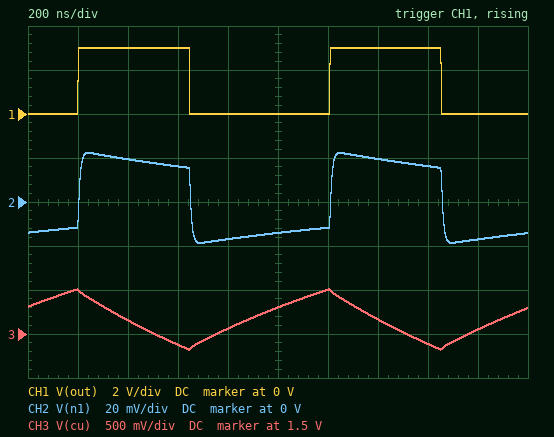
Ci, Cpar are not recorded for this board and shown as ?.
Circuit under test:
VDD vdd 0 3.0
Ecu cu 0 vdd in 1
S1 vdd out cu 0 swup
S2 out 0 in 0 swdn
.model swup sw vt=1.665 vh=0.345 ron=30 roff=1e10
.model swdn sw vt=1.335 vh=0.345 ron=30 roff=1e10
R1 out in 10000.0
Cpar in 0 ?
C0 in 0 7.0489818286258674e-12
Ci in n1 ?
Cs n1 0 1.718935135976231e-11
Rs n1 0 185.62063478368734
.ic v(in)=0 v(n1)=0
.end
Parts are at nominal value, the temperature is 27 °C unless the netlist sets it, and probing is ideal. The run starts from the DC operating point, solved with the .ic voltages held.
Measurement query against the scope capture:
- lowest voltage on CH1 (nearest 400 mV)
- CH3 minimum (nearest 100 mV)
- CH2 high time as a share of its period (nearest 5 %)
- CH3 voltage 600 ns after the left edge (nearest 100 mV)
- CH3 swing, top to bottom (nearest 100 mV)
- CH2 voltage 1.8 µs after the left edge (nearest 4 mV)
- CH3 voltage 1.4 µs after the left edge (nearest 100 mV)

0 V
1.3 V
45 %
1.4 V
700 mV
-16 mV
1.7 V
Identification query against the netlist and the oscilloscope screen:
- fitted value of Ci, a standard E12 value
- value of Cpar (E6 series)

68 pF
33 pF
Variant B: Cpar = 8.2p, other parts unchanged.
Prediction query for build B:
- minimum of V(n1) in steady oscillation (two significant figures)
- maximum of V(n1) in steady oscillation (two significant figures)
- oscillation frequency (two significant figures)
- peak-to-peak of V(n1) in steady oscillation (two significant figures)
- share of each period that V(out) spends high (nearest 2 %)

-24 mV
29 mV
1.3 MHz
53 mV
44 %
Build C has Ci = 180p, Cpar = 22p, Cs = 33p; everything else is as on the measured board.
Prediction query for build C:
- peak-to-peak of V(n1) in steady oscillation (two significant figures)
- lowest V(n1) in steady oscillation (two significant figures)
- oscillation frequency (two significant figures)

56 mV
-25 mV
520 kHz
